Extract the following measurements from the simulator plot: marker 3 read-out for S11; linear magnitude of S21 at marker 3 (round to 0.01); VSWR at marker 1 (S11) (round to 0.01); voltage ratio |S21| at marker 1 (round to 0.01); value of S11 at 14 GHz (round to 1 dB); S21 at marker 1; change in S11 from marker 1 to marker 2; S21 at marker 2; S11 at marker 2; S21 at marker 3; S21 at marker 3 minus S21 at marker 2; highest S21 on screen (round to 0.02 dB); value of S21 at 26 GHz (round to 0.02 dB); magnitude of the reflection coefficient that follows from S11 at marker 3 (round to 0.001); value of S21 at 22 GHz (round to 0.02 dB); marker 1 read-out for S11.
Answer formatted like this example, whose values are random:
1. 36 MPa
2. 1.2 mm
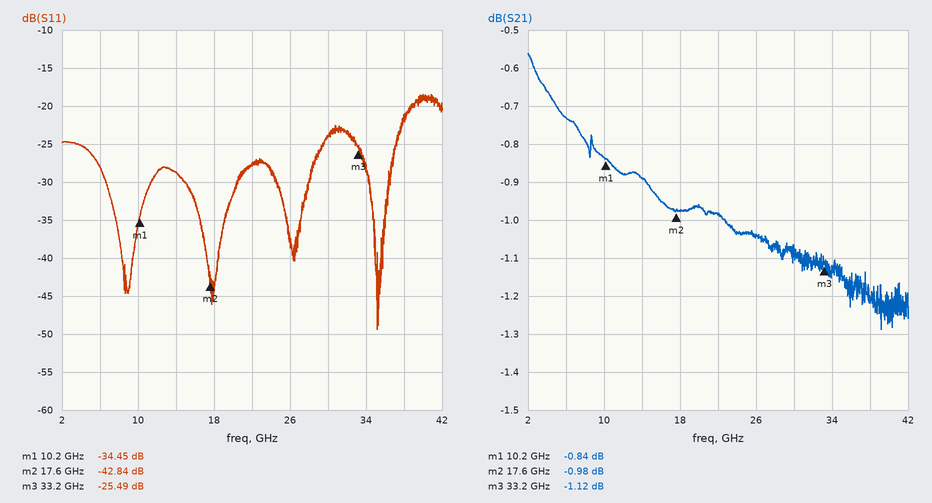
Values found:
1. -25.49 dB
2. 0.88
3. 1.04
4. 0.91
5. -29 dB
6. -0.84 dB
7. -8.39 dB
8. -0.98 dB
9. -42.84 dB
10. -1.12 dB
11. -0.14 dB
12. -0.56 dB
13. -1.04 dB
14. 0.053
15. -0.98 dB
16. -34.45 dB
